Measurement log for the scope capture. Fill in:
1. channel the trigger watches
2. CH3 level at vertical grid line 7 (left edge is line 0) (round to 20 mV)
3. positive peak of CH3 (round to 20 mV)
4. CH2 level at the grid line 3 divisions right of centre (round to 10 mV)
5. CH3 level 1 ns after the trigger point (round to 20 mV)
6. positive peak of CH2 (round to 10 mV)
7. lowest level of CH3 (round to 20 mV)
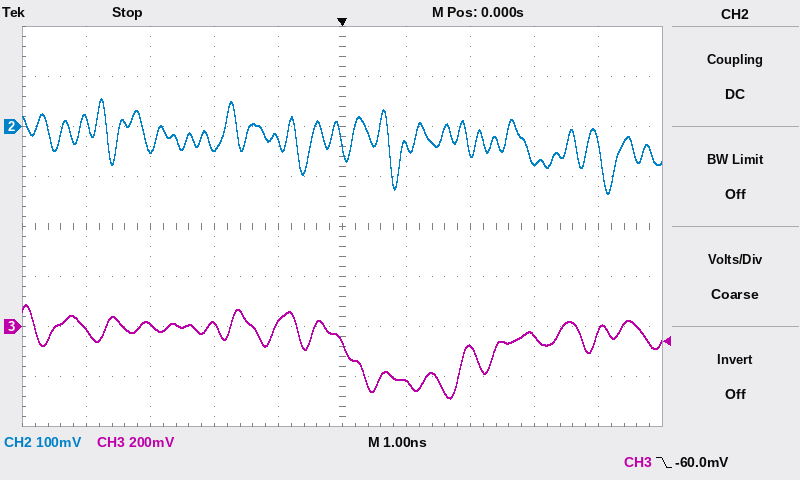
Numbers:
CH3
-80 mV
80 mV
-70 mV
-220 mV
60 mV
-280 mV
